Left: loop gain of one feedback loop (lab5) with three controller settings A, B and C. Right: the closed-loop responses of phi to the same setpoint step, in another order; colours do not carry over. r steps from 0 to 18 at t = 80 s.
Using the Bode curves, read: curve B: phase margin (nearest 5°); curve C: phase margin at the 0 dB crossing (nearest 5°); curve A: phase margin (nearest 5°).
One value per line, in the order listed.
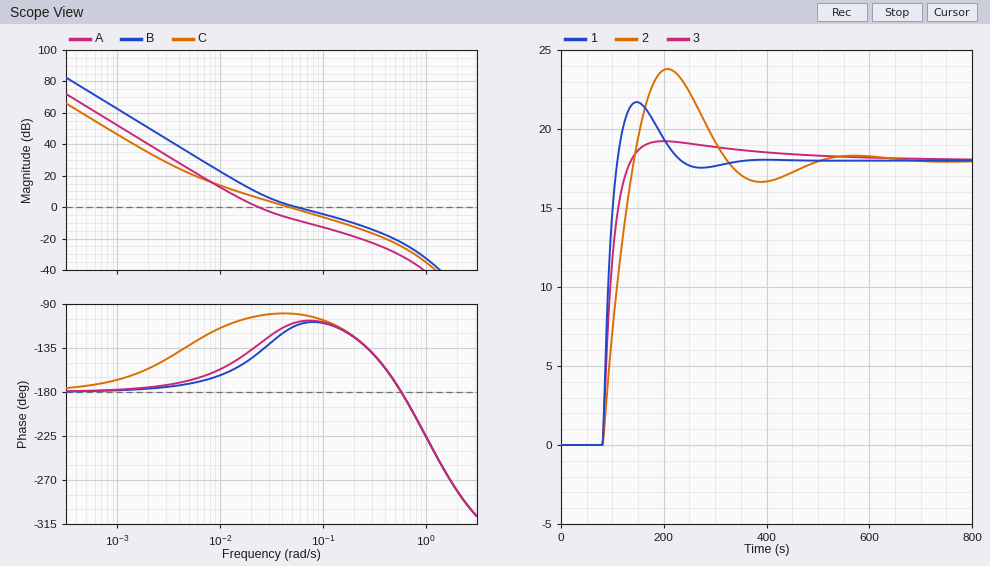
70°
80°
50°
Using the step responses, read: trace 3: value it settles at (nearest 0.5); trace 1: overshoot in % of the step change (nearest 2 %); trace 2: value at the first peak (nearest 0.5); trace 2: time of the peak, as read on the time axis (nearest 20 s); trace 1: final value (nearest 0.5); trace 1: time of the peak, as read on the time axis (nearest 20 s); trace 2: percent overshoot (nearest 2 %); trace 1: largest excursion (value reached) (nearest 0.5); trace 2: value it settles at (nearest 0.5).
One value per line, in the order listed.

18.0
20 %
24.0
200 s
18.0
140 s
32 %
21.5
18.0
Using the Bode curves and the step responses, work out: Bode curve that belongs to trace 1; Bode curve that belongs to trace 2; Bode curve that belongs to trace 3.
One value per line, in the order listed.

B
A
C
